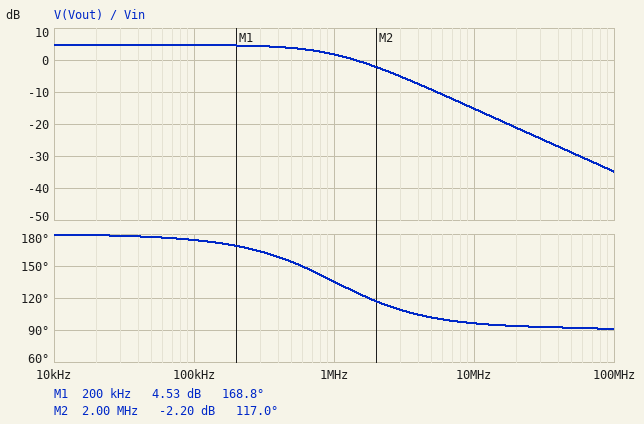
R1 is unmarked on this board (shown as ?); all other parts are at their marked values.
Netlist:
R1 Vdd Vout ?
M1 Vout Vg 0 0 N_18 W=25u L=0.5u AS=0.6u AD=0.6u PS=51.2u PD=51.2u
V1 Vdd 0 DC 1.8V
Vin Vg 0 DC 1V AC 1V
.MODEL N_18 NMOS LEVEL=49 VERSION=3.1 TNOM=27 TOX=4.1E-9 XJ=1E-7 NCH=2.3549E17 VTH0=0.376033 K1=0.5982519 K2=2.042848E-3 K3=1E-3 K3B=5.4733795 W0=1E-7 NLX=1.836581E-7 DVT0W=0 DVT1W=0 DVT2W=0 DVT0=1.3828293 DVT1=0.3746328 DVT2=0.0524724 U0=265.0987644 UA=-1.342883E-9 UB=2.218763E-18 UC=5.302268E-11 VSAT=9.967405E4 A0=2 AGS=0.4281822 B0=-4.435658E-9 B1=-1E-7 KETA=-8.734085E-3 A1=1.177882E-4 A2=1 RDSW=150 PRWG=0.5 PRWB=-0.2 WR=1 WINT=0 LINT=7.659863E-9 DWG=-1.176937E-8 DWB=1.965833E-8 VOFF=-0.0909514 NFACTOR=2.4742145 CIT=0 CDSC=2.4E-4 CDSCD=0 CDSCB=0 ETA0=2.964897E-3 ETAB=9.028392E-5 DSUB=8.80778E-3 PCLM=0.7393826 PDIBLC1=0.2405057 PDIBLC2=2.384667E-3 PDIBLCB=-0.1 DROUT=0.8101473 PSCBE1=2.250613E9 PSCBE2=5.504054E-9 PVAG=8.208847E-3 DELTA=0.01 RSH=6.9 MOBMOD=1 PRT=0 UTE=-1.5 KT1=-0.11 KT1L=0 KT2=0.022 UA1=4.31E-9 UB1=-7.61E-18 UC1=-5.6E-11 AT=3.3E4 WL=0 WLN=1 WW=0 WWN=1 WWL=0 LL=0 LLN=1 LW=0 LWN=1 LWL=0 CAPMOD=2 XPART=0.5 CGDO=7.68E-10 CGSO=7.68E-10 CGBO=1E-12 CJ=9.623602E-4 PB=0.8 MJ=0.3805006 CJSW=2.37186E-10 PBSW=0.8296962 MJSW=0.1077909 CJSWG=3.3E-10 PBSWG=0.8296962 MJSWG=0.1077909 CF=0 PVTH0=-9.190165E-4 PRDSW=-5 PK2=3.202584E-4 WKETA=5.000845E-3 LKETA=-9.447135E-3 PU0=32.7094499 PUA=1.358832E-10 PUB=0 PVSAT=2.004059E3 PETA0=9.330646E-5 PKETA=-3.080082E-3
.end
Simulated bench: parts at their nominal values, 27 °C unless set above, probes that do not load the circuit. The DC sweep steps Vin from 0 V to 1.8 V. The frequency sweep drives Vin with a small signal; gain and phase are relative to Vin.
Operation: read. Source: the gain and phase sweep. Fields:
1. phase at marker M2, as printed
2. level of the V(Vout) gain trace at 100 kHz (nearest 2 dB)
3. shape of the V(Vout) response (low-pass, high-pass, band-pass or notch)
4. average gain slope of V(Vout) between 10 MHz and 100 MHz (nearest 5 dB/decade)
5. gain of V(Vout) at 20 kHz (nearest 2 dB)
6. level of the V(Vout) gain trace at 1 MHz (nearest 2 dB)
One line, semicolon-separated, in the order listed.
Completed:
117.0 deg; 4 dB; low-pass; -20 dB/decade; 4 dB; 2 dB
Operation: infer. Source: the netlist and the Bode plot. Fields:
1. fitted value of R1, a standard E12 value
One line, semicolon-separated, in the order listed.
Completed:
390 Ω
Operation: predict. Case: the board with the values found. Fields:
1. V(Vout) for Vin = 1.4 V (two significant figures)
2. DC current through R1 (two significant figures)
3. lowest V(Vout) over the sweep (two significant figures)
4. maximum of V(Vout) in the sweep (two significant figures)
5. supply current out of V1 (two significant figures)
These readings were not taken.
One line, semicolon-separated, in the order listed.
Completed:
550 mV; 1.4 mA; 380 mV; 1.8 V; 1.4 mA
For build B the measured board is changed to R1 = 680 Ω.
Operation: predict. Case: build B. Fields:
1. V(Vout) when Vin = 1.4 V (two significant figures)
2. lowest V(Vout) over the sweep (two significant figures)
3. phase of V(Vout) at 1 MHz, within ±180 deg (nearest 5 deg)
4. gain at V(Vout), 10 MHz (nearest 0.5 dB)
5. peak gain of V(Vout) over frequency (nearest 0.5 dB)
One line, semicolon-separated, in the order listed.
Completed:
290 mV; 220 mV; 120 deg; -16.0 dB; 9.0 dB
